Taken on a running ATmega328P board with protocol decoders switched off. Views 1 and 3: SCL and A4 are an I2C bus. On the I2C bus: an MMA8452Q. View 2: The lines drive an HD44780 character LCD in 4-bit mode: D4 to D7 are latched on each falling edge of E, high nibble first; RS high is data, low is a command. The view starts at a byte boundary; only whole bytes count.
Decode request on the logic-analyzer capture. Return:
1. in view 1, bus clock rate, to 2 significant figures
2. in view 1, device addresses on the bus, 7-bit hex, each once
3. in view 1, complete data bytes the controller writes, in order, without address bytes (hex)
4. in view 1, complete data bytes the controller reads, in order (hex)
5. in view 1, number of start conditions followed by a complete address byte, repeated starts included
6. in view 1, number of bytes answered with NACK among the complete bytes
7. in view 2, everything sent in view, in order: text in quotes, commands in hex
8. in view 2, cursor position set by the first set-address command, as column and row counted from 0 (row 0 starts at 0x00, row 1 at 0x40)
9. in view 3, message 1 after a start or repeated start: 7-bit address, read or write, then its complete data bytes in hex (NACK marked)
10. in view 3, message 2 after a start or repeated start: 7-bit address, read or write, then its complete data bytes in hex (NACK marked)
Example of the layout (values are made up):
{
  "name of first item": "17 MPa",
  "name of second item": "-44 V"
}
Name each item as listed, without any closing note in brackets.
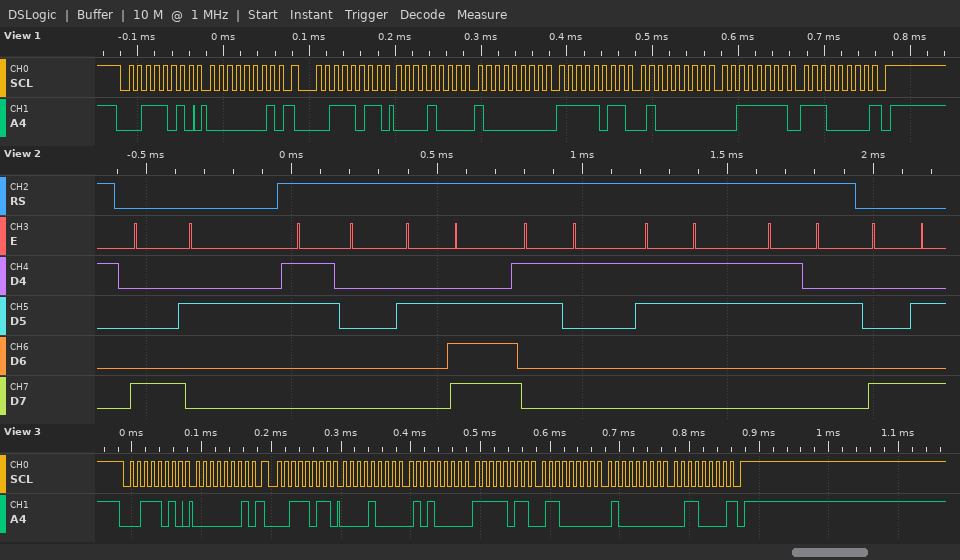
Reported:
{
  "in view 1, bus clock rate, to 2 significant figures": "100 kHz",
  "in view 1, device addresses on the bus, 7-bit hex, each once": "0x1D",
  "in view 1, complete data bytes the controller writes, in order, without address bytes": "01",
  "in view 1, complete data bytes the controller reads, in order": "08 80 FB 40 3F E0",
  "in view 1, number of start conditions followed by a complete address byte, repeated starts included": "2",
  "in view 1, number of bytes answered with NACK among the complete bytes": "1",
  "in view 2, everything sent in view, in order: text in quotes, commands in hex": "0x82 \"0.132\" 0x8A",
  "in view 2, cursor position set by the first set-address command, as column and row counted from 0": "column 2, row 0",
  "in view 3, message 1 after a start or repeated start: 7-bit address, read or write, then its complete data bytes in hex": "0x1D write: 01",
  "in view 3, message 2 after a start or repeated start: 7-bit address, read or write, then its complete data bytes in hex": "0x1D read: 08 50 FB 60 40 30 NACK"
}
